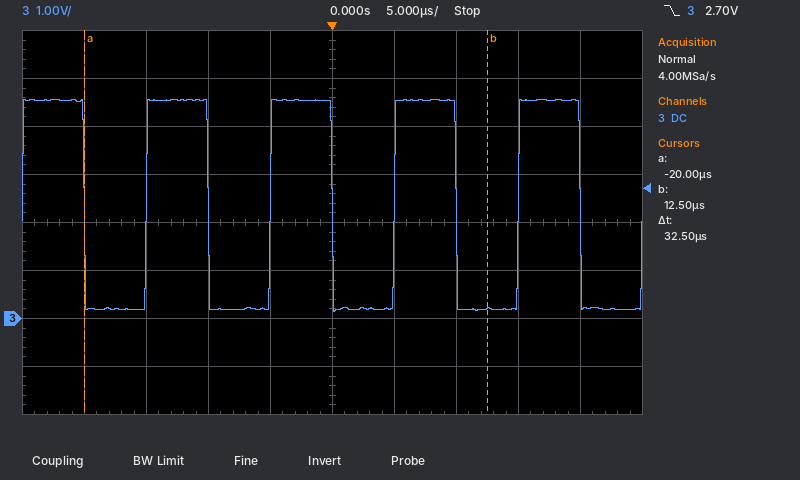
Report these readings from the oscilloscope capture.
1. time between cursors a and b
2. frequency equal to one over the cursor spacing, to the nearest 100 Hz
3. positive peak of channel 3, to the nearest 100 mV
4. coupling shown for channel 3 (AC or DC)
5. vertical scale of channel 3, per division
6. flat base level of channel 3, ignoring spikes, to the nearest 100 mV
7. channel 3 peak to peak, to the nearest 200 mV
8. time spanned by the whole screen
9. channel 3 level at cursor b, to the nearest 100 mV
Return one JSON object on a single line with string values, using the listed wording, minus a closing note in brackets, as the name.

{"time between cursors a and b": "32.5 µs", "frequency equal to one over the cursor spacing, to the nearest 100 Hz": "30.8 kHz", "positive peak of channel 3, to the nearest 100 mV": "4.6 V", "coupling shown for channel 3": "DC", "vertical scale of channel 3, per division": "1 V", "flat base level of channel 3, ignoring spikes, to the nearest 100 mV": "200 mV", "channel 3 peak to peak, to the nearest 200 mV": "4.4 V", "time spanned by the whole screen": "50 µs", "channel 3 level at cursor b, to the nearest 100 mV": "200 mV"}
